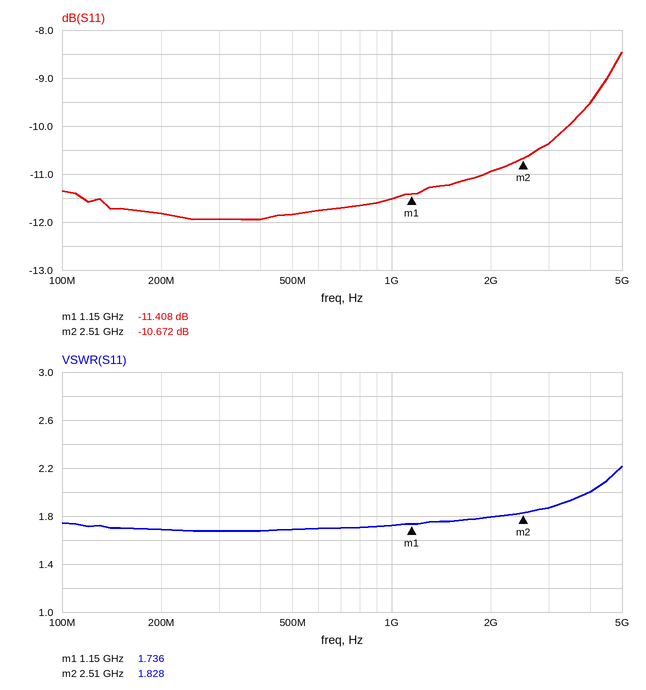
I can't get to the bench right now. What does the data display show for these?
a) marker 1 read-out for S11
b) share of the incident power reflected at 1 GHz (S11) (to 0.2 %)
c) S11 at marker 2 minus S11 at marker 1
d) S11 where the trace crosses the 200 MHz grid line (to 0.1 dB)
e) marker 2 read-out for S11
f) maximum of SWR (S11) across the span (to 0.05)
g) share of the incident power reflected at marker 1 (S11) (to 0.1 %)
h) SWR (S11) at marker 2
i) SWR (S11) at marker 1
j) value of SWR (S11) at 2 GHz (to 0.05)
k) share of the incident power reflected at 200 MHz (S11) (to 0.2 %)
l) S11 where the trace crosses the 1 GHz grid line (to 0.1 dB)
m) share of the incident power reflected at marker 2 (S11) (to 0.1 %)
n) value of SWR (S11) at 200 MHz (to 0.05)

-11.408 dB
7.0 %
0.736 dB
-11.8 dB
-10.672 dB
2.20
7.2 %
1.828
1.736
1.80
6.6 %
-11.5 dB
8.6 %
1.70
